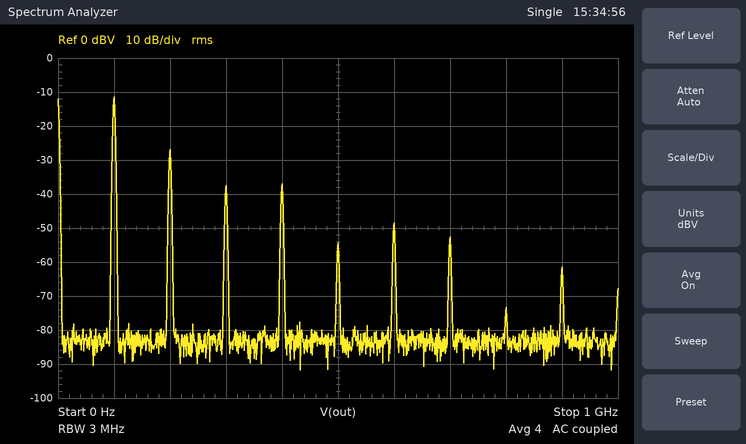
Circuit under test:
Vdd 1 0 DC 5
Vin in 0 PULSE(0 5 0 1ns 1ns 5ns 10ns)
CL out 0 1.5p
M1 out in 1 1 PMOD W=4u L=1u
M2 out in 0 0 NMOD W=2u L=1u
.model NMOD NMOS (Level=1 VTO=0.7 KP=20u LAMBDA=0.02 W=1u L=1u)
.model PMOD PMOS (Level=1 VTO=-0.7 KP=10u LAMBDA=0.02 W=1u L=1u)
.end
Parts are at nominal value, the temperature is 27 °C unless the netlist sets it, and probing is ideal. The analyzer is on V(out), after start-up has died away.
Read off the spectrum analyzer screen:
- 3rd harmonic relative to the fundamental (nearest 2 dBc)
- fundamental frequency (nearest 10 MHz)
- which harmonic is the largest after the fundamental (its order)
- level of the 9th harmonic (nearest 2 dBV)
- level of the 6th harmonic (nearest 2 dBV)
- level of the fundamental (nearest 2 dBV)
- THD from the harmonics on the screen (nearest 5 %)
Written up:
-26 dBc
100 MHz
2
-62 dBV
-48 dBV
-12 dBV
20 %
